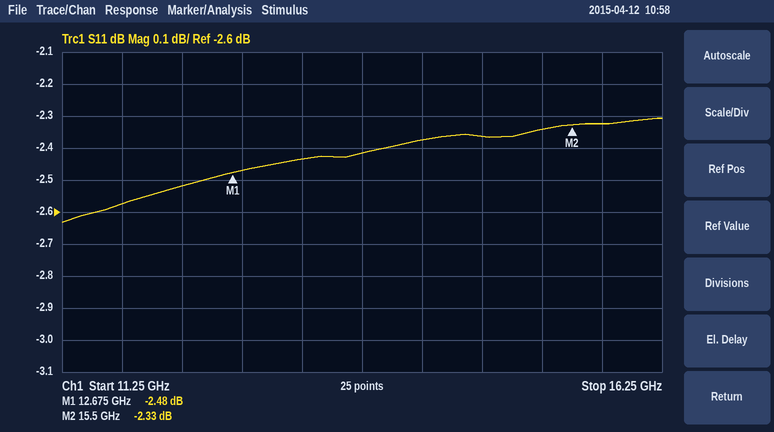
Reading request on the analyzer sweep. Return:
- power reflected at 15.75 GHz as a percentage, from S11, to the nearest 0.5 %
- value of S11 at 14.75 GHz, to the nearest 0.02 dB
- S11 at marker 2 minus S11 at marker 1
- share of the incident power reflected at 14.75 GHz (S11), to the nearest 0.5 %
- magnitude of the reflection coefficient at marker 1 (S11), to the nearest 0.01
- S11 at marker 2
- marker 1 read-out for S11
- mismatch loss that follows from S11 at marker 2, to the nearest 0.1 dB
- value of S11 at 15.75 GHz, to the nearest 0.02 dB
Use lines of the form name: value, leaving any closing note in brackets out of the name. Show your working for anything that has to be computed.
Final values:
power reflected at 15.75 GHz as a percentage, from S11, to the nearest 0.5 %: 10^(-2.32/10) ≈ 58.6 %, so 58.5 % to the nearest 0.5 %
value of S11 at 14.75 GHz, to the nearest 0.02 dB: -2.36 dB
S11 at marker 2 minus S11 at marker 1: -2.33 − (-2.48) = 0.15 dB
share of the incident power reflected at 14.75 GHz (S11), to the nearest 0.5 %: 10^(-2.36/10) ≈ 58.1 %, so 58.0 % to the nearest 0.5 %
magnitude of the reflection coefficient at marker 1 (S11), to the nearest 0.01: 10^(-2.48/20) ≈ 0.75
S11 at marker 2: -2.33 dB
marker 1 read-out for S11: -2.48 dB
mismatch loss that follows from S11 at marker 2, to the nearest 0.1 dB: −10 log10(1 − 10^(-2.33/10)) ≈ 3.8 dB
value of S11 at 15.75 GHz, to the nearest 0.02 dB: -2.32 dB
